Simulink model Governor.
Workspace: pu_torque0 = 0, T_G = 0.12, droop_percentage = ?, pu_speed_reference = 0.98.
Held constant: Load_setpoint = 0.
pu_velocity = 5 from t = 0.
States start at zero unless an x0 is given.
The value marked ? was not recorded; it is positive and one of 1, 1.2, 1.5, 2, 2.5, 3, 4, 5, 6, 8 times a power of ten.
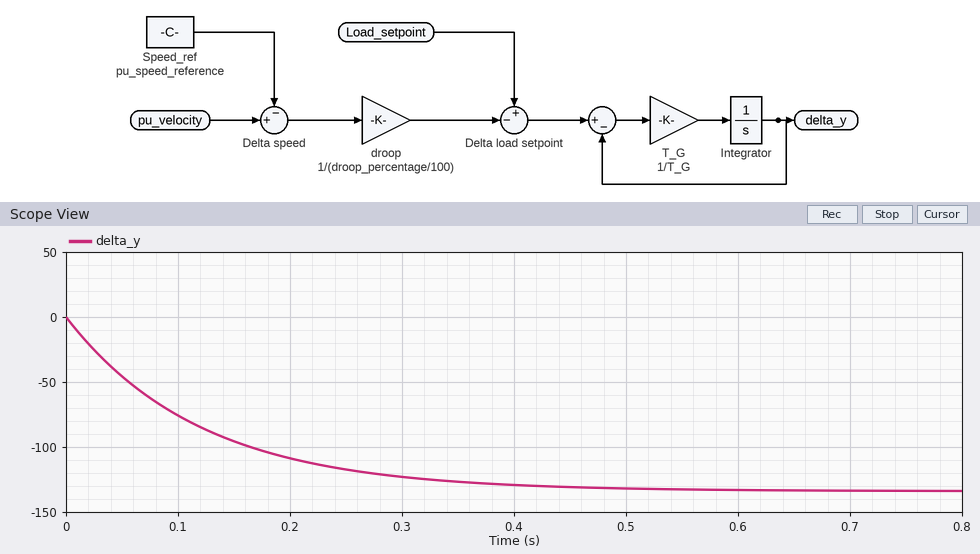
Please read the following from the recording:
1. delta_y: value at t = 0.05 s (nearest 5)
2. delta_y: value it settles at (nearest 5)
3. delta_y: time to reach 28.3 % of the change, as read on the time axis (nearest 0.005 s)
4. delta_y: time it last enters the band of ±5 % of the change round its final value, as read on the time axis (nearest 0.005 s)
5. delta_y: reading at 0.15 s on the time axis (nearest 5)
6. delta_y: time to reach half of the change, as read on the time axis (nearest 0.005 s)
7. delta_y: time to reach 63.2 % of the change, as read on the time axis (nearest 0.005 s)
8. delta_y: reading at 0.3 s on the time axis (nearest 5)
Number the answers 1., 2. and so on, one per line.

1. -45
2. -135
3. 0.040 s
4. 0.360 s
5. -95
6. 0.085 s
7. 0.120 s
8. -125
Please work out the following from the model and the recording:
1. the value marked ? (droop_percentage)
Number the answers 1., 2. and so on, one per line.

1. 3
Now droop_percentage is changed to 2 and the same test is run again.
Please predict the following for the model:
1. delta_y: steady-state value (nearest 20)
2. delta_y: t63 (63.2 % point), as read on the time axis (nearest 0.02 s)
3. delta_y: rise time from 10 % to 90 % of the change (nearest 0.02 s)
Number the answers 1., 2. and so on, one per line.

1. -200
2. 0.12 s
3. 0.26 s
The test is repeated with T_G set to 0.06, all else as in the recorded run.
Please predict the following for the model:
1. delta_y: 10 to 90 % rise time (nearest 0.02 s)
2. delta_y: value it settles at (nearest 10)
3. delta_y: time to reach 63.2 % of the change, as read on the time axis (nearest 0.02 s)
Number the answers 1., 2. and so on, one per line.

1. 0.14 s
2. -130
3. 0.06 s
